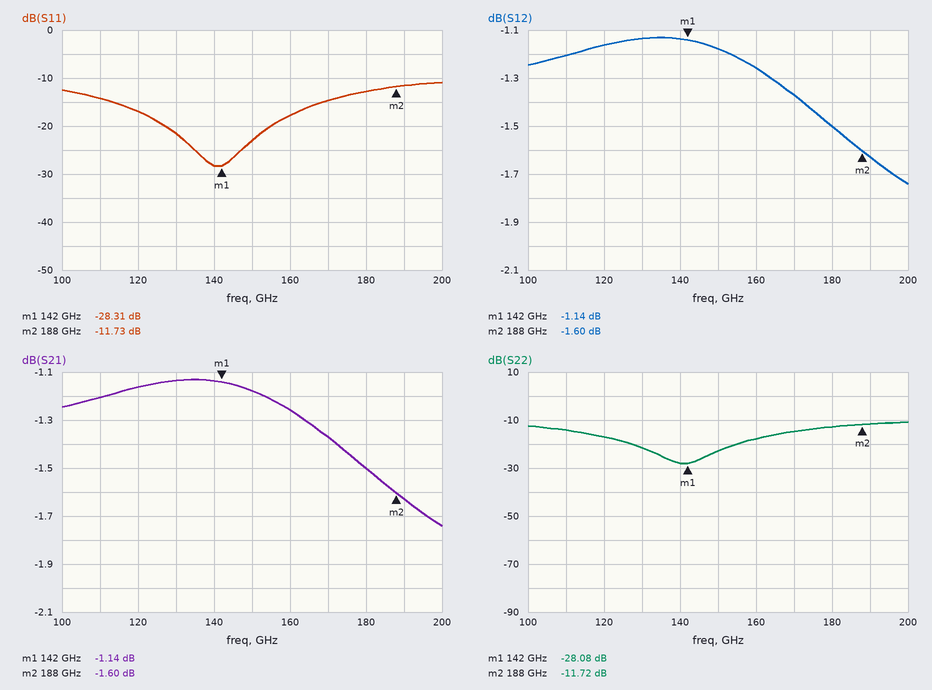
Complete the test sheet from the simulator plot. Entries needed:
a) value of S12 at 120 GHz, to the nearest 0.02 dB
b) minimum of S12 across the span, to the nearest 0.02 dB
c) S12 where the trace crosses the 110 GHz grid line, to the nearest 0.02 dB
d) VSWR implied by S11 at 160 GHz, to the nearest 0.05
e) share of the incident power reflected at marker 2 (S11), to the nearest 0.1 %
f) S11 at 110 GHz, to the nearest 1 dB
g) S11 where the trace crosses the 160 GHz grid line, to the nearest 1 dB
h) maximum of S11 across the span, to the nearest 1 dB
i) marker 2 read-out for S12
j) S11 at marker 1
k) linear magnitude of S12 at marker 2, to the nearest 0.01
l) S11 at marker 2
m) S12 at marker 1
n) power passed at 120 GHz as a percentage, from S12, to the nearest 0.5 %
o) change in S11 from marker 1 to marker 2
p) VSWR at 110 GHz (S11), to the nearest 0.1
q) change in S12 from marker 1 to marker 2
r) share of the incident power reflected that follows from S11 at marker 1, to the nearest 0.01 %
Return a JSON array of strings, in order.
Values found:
["-1.16 dB", "-1.74 dB", "-1.20 dB", "1.30", "6.7 %", "-14 dB", "-18 dB", "-11 dB", "-1.60 dB", "-28.31 dB", "0.83", "-11.73 dB", "-1.14 dB", "76.5 %", "16.58 dB", "1.5", "-0.46 dB", "0.15 %"]
